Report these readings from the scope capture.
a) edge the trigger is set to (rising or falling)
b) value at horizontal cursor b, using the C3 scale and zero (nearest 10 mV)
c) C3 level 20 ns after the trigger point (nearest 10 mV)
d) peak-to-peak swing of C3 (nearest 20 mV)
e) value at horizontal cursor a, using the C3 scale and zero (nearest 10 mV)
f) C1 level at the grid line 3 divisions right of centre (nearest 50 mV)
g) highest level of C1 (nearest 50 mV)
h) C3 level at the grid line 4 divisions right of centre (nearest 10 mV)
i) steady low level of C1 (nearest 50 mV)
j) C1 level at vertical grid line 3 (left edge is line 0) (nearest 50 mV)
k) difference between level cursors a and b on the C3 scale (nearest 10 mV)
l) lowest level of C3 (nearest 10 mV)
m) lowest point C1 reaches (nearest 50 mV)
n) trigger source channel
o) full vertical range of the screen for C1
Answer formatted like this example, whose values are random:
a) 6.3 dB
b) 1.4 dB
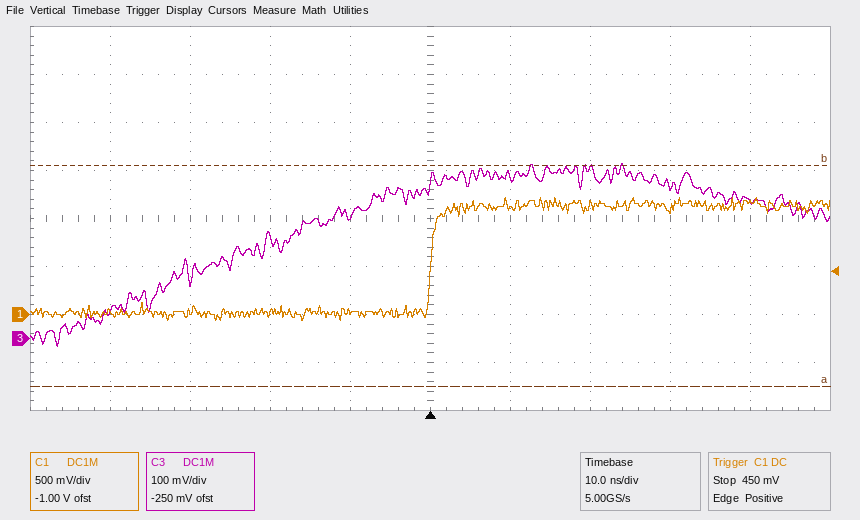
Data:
a) rising
b) 360 mV
c) 350 mV
d) 380 mV
e) -100 mV
f) 1.10 V
g) 1.20 V
h) 290 mV
i) 0 mV
j) 0 mV
k) 460 mV
l) -20 mV
m) -50 mV
n) C1
o) 4 V
